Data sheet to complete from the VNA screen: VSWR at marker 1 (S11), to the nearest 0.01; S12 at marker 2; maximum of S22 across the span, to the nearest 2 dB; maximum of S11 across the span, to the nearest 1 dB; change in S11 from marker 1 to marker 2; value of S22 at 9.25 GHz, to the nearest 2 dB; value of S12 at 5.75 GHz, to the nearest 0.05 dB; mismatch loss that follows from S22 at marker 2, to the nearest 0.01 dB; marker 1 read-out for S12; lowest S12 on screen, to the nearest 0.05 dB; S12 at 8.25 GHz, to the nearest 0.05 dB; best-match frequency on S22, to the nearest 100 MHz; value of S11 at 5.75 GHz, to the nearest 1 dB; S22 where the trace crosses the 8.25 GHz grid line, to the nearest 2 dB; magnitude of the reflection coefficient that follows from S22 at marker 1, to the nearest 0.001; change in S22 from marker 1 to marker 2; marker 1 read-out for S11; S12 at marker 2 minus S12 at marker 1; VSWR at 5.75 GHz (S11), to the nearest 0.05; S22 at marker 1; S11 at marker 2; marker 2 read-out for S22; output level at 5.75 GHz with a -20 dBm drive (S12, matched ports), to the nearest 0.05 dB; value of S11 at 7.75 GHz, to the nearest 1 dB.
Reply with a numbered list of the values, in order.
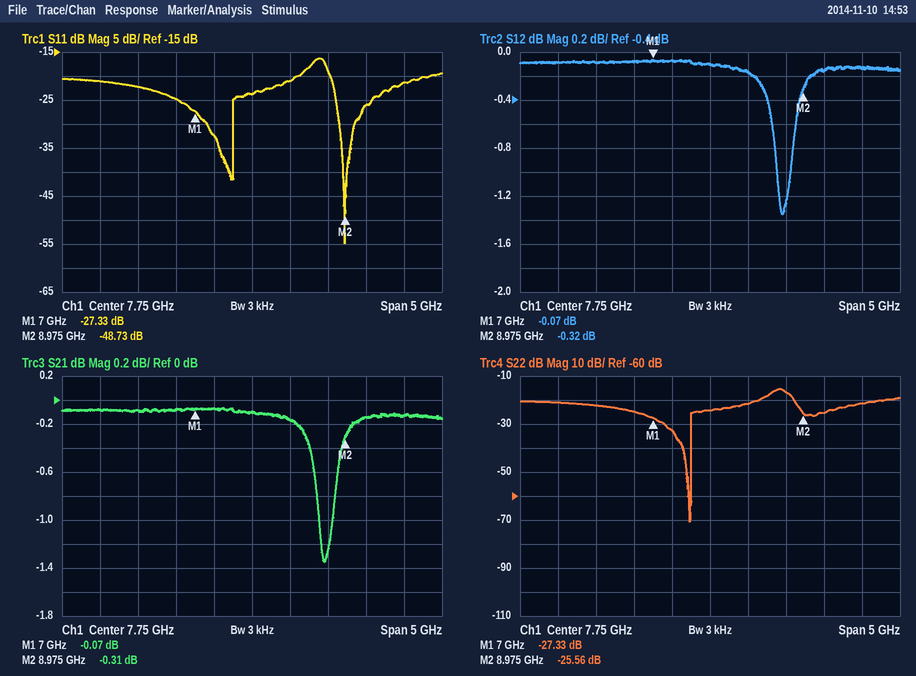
1. 1.09
2. -0.32 dB
3. -16 dB
4. -16 dB
5. -21.40 dB
6. -26 dB
7. -0.10 dB
8. 0.01 dB
9. -0.07 dB
10. -1.35 dB
11. -0.15 dB
12. 7.5 GHz
13. -21 dB
14. -22 dB
15. 0.043
16. 1.77 dB
17. -27.33 dB
18. -0.25 dB
19. 1.20
20. -27.33 dB
21. -48.73 dB
22. -25.56 dB
23. -20.10 dBm
24. -24 dB
